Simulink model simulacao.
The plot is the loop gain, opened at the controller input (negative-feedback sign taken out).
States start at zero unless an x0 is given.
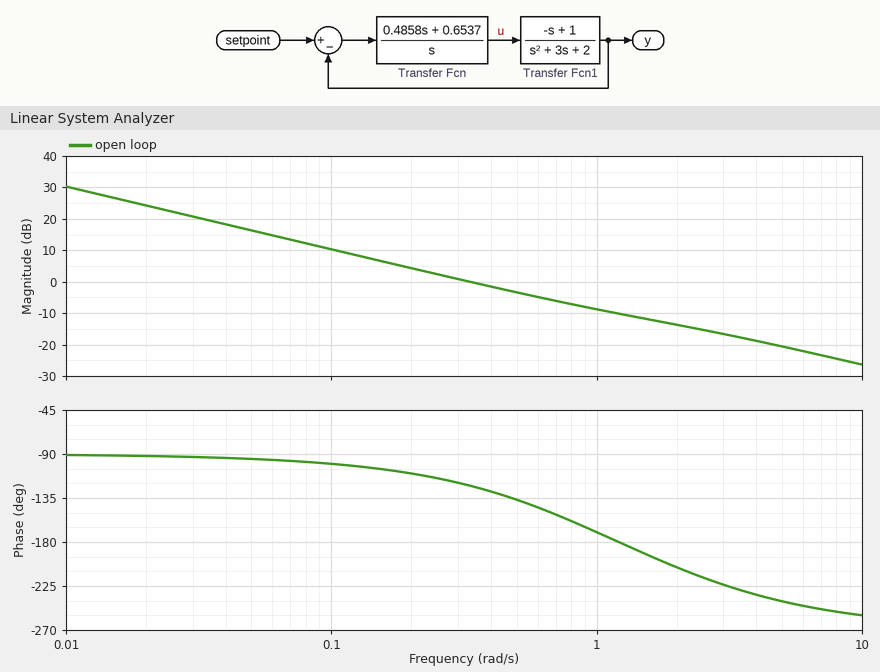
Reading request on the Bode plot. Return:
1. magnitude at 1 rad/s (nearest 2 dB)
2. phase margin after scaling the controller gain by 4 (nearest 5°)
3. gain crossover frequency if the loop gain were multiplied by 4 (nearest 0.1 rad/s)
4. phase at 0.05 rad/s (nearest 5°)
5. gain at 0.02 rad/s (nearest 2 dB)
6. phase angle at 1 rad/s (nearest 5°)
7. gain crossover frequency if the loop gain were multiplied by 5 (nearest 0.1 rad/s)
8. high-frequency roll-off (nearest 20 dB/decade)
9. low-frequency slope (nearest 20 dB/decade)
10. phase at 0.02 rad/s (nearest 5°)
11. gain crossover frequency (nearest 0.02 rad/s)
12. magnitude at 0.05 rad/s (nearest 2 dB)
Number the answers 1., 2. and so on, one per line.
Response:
1. -8 dB
2. -15°
3. 1.6 rad/s
4. -95°
5. 24 dB
6. -170°
7. 2.1 rad/s
8. -20 dB/decade
9. -20 dB/decade
10. -90°
11. 0.34 rad/s
12. 16 dB
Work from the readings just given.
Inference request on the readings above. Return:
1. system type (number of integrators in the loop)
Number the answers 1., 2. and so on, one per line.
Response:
1. 1
